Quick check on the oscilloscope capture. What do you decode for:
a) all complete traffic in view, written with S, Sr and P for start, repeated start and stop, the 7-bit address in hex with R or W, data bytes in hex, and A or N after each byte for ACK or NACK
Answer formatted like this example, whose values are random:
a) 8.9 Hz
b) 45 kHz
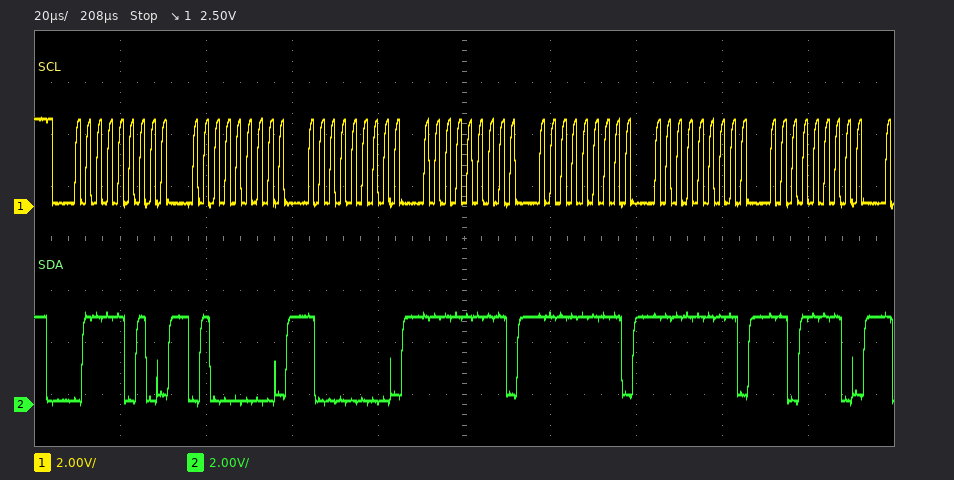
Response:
a) S 3DW A 40 A 80 A FF A FF A FF A DE A
